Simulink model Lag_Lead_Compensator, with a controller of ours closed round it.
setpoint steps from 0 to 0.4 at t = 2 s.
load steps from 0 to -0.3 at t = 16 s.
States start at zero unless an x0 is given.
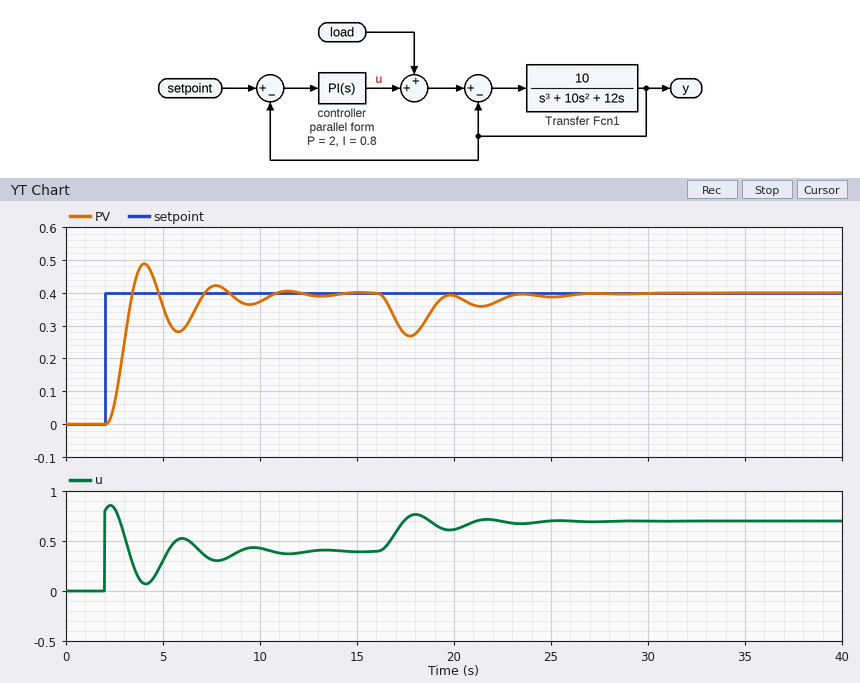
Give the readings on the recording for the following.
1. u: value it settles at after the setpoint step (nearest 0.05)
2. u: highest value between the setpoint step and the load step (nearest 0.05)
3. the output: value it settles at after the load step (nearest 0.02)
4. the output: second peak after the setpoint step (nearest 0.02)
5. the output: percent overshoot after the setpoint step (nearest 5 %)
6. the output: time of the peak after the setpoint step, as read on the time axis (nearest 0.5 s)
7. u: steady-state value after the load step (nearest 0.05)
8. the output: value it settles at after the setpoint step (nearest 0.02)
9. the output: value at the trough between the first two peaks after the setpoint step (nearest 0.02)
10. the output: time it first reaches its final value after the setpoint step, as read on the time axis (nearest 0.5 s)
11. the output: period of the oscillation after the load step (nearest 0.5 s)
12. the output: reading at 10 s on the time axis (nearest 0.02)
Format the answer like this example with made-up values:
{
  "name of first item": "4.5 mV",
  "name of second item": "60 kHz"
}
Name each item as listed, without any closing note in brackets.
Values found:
{
  "u: value it settles at after the setpoint step": "0.40",
  "u: highest value between the setpoint step and the load step": "0.85",
  "the output: value it settles at after the load step": "0.40",
  "the output: second peak after the setpoint step": "0.42",
  "the output: percent overshoot after the setpoint step": "20 %",
  "the output: time of the peak after the setpoint step, as read on the time axis": "4.0 s",
  "u: steady-state value after the load step": "0.70",
  "the output: value it settles at after the setpoint step": "0.40",
  "the output: value at the trough between the first two peaks after the setpoint step": "0.28",
  "the output: time it first reaches its final value after the setpoint step, as read on the time axis": "3.5 s",
  "the output: period of the oscillation after the load step": "3.5 s",
  "the output: reading at 10 s on the time axis": "0.38"
}
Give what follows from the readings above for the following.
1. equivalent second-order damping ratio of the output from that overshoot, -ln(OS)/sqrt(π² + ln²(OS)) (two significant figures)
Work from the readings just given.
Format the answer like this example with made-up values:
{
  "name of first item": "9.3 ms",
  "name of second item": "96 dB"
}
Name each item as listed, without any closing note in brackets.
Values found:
{
  "equivalent second-order damping ratio of the output from that overshoot, -ln(OS)/sqrt(π² + ln²(OS))": "0.46"
}
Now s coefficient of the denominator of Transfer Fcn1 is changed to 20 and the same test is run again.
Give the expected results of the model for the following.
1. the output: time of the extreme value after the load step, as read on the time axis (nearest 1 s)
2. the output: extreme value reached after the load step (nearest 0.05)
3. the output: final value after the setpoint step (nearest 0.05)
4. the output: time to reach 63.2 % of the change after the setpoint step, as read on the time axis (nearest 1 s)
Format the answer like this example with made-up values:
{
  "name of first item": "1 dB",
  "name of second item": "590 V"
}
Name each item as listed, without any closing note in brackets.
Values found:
{
  "the output: time of the extreme value after the load step, as read on the time axis": "18 s",
  "the output: extreme value reached after the load step": "0.30",
  "the output: final value after the setpoint step": "0.40",
  "the output: time to reach 63.2 % of the change after the setpoint step, as read on the time axis": "3 s"
}
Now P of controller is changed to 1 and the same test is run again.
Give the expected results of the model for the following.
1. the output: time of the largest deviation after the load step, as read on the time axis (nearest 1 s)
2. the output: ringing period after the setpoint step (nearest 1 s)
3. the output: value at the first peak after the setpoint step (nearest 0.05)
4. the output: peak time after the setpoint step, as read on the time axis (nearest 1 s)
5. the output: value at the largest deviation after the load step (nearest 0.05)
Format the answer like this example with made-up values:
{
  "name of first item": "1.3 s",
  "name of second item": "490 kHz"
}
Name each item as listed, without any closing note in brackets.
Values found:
{
  "the output: time of the largest deviation after the load step, as read on the time axis": "18 s",
  "the output: ringing period after the setpoint step": "5 s",
  "the output: value at the first peak after the setpoint step": "0.45",
  "the output: peak time after the setpoint step, as read on the time axis": "5 s",
  "the output: value at the largest deviation after the load step": "0.25"
}
